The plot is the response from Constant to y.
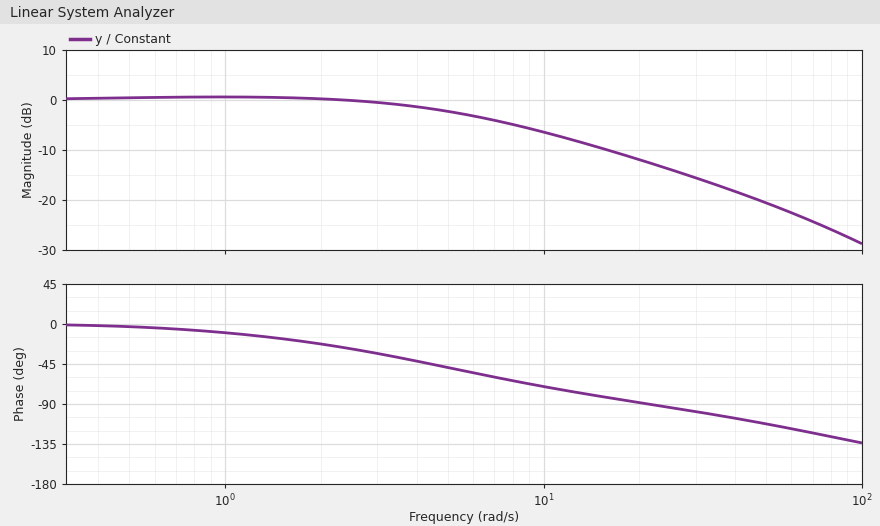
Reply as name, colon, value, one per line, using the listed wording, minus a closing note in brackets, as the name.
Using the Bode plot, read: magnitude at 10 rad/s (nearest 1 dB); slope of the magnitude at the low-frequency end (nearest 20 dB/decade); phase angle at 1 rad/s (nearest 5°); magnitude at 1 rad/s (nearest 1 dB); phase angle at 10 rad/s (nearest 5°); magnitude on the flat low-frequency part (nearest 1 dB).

magnitude at 10 rad/s: -6 dB
slope of the magnitude at the low-frequency end: 0 dB/decade
phase angle at 1 rad/s: -10°
magnitude at 1 rad/s: 1 dB
phase angle at 10 rad/s: -70°
magnitude on the flat low-frequency part: 0 dB
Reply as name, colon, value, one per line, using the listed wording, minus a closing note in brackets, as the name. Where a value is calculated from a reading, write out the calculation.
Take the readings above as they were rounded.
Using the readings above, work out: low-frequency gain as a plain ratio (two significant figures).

low-frequency gain as a plain ratio: 10^(0 / 20) = 1.0
